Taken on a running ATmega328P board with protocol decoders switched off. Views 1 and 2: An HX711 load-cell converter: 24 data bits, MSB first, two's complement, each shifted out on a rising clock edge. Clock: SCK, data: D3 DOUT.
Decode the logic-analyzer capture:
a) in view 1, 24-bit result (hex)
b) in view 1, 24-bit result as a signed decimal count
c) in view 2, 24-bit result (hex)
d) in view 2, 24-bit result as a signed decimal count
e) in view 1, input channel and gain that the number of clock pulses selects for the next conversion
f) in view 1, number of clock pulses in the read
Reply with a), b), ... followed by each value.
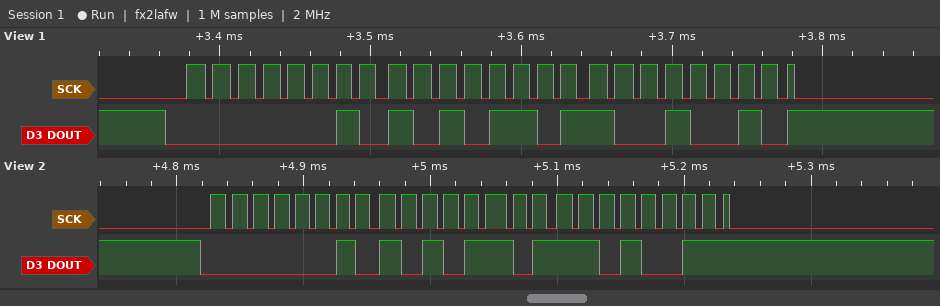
a) 0x02AD92
b) 175506
c) 0x02ADD3
d) 175571
e) channel A, gain 128
f) 25
